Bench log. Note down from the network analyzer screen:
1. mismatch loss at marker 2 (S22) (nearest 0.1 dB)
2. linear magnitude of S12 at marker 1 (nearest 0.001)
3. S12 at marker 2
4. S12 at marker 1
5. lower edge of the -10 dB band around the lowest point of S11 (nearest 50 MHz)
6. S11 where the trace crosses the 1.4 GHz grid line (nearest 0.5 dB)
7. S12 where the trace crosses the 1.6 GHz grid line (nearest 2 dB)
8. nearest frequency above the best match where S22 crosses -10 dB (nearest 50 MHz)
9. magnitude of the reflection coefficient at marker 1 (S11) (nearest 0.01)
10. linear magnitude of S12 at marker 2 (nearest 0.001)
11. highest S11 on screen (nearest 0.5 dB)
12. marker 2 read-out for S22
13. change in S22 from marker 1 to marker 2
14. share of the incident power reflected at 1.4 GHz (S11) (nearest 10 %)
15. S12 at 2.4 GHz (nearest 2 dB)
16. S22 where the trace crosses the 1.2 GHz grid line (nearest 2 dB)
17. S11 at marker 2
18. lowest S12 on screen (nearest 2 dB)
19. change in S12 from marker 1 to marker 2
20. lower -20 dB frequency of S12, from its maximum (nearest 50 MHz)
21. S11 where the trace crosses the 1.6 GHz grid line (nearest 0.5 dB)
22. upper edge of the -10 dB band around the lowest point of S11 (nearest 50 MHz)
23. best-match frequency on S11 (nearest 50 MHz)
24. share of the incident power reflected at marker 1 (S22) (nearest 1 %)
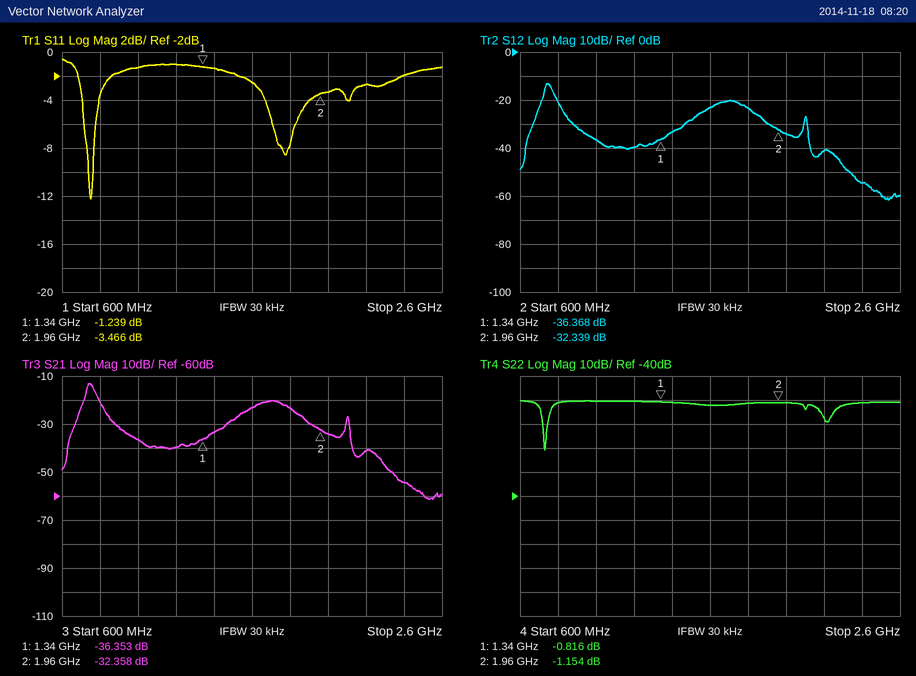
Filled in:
6.3 dB
0.015
-32.339 dB
-36.368 dB
750 MHz
-1.5 dB
-24 dB
750 MHz
0.87
0.024
-0.5 dB
-1.154 dB
-0.338 dB
70 %
-54 dB
0 dB
-3.466 dB
-62 dB
4.029 dB
650 MHz
-2.5 dB
750 MHz
750 MHz
83 %
